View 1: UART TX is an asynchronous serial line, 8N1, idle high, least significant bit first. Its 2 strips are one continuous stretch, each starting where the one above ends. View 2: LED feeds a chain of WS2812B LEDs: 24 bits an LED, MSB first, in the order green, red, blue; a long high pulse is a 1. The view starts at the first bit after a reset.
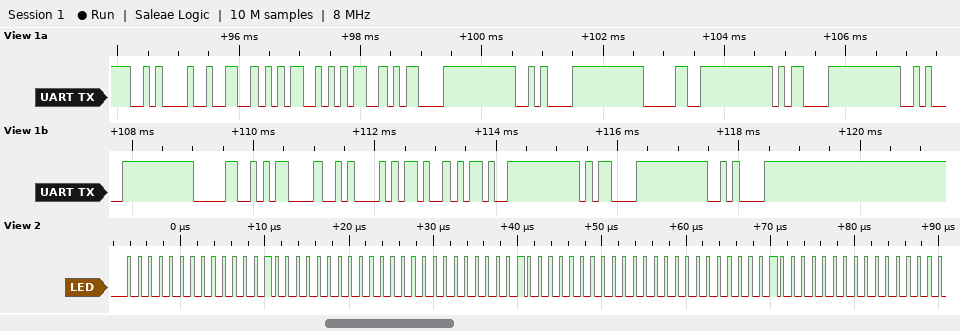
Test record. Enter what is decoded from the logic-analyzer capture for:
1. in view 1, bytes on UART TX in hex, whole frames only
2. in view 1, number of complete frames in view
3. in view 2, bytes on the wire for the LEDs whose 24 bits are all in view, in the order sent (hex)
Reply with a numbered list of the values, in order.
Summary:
1. 0x0A 0x32 0x35 0x35 0x0D 0x0A 0x30 0x0D 0x0A 0x30 0x0D 0x0A 0x2D 0x2D 0x0D 0x0A
2. 16
3. 00 04 00 00 04 00 00 04 00
